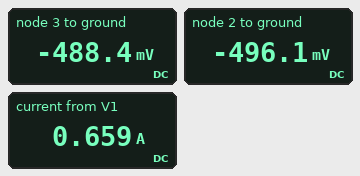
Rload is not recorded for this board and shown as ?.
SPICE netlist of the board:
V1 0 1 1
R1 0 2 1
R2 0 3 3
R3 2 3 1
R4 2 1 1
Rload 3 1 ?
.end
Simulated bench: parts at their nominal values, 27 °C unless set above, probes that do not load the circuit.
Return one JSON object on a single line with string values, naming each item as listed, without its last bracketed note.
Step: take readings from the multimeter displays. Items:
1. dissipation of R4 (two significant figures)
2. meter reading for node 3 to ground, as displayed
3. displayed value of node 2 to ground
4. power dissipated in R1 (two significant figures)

{"dissipation of R4": "250 mW", "meter reading for node 3 to ground, as displayed": "-488.4 mV", "displayed value of node 2 to ground": "-496.1 mV", "power dissipated in R1": "250 mW"}
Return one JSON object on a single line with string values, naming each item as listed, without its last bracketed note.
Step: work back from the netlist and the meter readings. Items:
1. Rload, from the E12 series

{"Rload, from the E12 series": "3.3 Ω"}
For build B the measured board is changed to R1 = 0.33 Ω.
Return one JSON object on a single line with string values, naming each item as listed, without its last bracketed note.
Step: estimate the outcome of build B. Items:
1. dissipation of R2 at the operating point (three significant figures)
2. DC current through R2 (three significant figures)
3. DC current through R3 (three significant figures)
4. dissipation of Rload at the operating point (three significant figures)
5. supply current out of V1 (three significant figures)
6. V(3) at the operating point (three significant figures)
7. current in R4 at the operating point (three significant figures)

{"dissipation of R2 at the operating point": "40.6 mW", "DC current through R2": "116 mA", "DC current through R3": "80.9 mA", "dissipation of Rload at the operating point": "128 mW", "supply current out of V1": "929 mA", "V(3) at the operating point": "-349 mV", "current in R4 at the operating point": "732 mA"}
